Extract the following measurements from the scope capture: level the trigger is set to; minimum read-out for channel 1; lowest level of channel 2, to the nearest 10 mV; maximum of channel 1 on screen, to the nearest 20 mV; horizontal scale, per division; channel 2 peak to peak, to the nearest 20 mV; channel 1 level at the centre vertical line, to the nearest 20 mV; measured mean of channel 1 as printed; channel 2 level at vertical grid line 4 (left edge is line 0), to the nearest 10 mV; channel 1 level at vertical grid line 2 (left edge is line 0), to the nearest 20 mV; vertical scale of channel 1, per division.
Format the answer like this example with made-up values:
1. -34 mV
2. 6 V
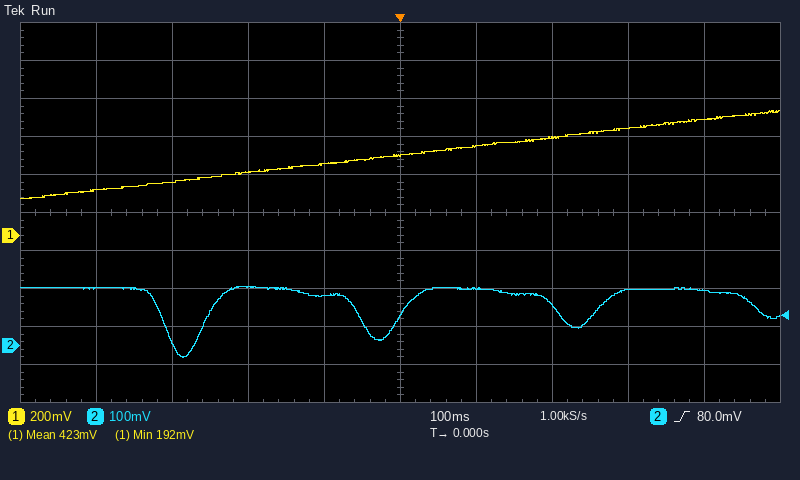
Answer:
1. 80.0 mV
2. 192 mV
3. -30 mV
4. 660 mV
5. 100 ms
6. 180 mV
7. 420 mV
8. 423 mV
9. 130 mV
10. 280 mV
11. 200 mV
